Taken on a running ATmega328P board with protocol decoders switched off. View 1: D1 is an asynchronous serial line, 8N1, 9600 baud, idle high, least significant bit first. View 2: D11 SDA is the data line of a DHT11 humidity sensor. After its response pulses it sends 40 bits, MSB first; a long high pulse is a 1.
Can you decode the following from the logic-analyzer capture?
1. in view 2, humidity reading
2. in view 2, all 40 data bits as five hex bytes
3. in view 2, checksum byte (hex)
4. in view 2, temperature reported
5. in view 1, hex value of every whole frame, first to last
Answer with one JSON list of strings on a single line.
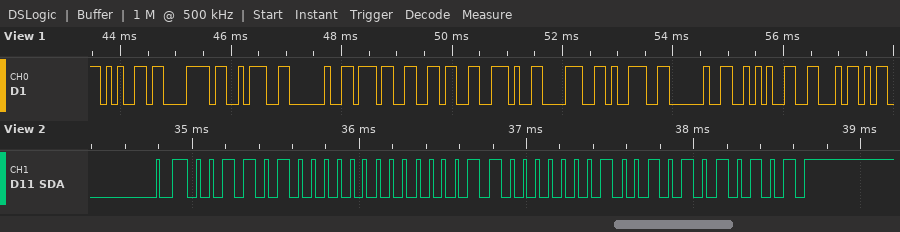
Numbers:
["52 %", "34 00 18 09 55", "0x55", "24.9 °C", "65 78 3A 20 37 36 2E 38 39 20 2A 46"]
